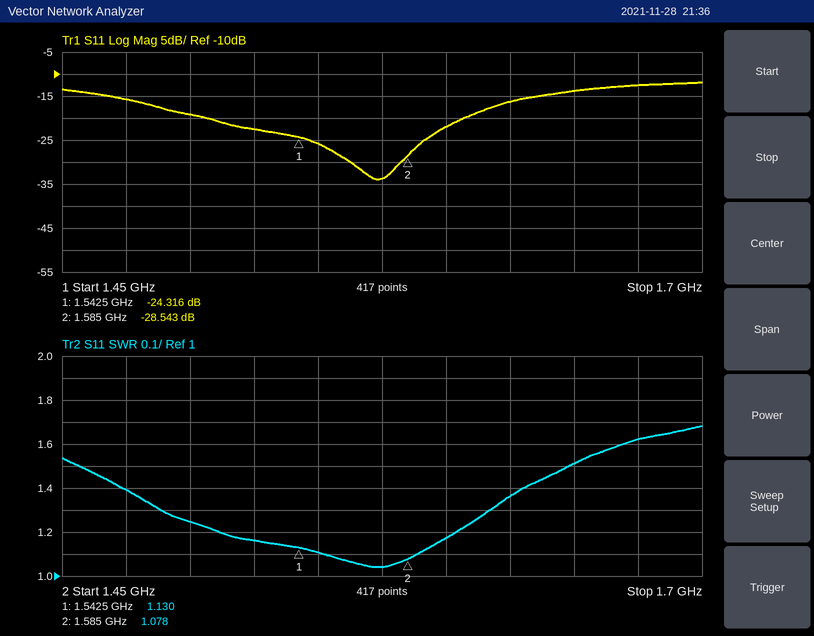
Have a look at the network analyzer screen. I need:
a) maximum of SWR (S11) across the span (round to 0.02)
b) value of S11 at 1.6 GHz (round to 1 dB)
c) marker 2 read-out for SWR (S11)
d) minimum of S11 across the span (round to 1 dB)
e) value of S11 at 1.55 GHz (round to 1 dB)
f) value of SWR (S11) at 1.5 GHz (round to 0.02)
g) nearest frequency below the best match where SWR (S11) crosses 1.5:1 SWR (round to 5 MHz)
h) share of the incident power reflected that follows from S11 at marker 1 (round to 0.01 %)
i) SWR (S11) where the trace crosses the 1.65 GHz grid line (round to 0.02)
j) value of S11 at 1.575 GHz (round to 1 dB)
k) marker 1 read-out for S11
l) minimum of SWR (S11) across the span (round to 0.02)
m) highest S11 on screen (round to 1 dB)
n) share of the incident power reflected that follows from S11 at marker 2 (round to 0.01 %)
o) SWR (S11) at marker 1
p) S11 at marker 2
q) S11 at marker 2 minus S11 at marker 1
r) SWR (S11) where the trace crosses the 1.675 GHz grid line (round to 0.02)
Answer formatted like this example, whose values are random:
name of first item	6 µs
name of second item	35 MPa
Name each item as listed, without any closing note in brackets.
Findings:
maximum of SWR (S11) across the span	1.68
value of S11 at 1.6 GHz	-22 dB
marker 2 read-out for SWR	1.078
minimum of S11 across the span	-34 dB
value of S11 at 1.55 GHz	-26 dB
value of SWR (S11) at 1.5 GHz	1.24
nearest frequency below the best match where SWR (S11) crosses 1.5:1 SWR	1.455 GHz
share of the incident power reflected that follows from S11 at marker 1	0.37 %
SWR (S11) where the trace crosses the 1.65 GHz grid line	1.52
value of S11 at 1.575 GHz	-34 dB
marker 1 read-out for S11	-24.316 dB
minimum of SWR (S11) across the span	1.04
highest S11 on screen	-12 dB
share of the incident power reflected that follows from S11 at marker 2	0.14 %
SWR (S11) at marker 1	1.130
S11 at marker 2	-28.543 dB
S11 at marker 2 minus S11 at marker 1	-4.227 dB
SWR (S11) where the trace crosses the 1.675 GHz grid line	1.62
